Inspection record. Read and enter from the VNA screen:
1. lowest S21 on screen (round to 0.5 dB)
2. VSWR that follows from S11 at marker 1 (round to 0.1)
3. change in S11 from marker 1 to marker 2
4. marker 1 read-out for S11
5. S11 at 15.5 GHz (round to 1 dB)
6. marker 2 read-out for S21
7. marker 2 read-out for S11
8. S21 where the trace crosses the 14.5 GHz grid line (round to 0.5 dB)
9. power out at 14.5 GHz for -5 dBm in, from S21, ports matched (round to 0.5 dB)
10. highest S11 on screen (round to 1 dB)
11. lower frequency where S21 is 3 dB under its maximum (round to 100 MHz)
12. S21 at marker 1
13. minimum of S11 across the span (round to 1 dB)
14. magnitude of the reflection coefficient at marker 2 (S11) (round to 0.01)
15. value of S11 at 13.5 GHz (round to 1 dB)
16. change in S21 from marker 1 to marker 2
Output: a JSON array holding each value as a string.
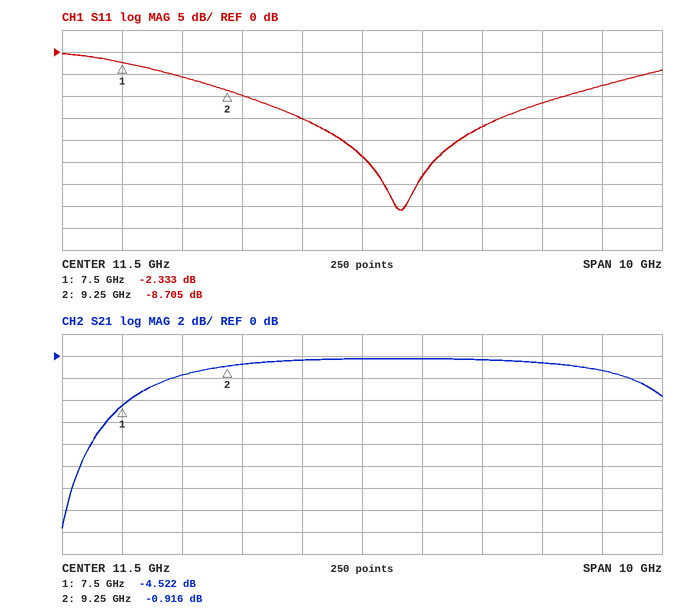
["-15.5 dB", "7.5", "-6.372 dB", "-2.333 dB", "-8 dB", "-0.916 dB", "-8.705 dB", "-0.5 dB", "-5.5 dBm", "0 dB", "7.8 GHz", "-4.522 dB", "-36 dB", "0.37", "-17 dB", "3.606 dB"]
